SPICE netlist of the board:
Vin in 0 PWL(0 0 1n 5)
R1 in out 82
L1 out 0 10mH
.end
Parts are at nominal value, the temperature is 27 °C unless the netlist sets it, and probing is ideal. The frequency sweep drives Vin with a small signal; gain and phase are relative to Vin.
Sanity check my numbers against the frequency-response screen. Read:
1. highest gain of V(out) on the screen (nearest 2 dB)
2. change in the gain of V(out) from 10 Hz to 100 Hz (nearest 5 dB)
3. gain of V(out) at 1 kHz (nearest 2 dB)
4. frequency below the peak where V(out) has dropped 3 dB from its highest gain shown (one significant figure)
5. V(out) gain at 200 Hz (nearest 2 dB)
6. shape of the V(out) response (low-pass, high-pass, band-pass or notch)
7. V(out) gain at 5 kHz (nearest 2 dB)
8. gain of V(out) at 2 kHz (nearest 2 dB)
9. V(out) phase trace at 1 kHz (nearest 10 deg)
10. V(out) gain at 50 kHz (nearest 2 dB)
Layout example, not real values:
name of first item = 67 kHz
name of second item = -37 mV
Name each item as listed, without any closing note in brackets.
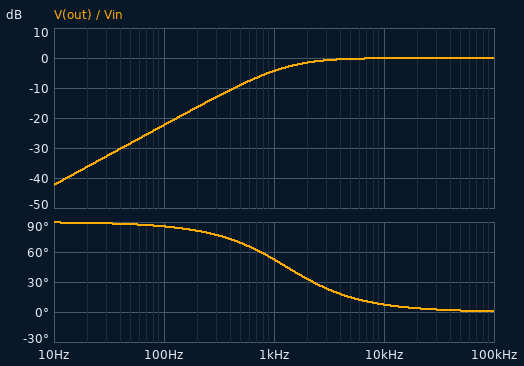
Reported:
highest gain of V(out) on the screen = 0 dB
change in the gain of V(out) from 10 Hz to 100 Hz = 20 dB
gain of V(out) at 1 kHz = -4 dB
frequency below the peak where V(out) has dropped 3 dB from its highest gain shown = 1 kHz
V(out) gain at 200 Hz = -16 dB
shape of the V(out) response = high-pass
V(out) gain at 5 kHz = 0 dB
gain of V(out) at 2 kHz = -2 dB
V(out) phase trace at 1 kHz = 50 deg
V(out) gain at 50 kHz = 0 dB
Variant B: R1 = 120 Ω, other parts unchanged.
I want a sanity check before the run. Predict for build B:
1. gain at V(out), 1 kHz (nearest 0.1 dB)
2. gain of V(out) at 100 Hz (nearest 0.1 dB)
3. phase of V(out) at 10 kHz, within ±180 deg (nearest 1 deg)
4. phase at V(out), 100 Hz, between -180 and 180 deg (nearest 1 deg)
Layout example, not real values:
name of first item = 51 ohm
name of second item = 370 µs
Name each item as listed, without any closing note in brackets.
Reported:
gain at V(out), 1 kHz = -6.7 dB
gain of V(out) at 100 Hz = -25.6 dB
phase of V(out) at 10 kHz, within ±180 deg = 11 deg
phase at V(out), 100 Hz, between -180 and 180 deg = 87 deg
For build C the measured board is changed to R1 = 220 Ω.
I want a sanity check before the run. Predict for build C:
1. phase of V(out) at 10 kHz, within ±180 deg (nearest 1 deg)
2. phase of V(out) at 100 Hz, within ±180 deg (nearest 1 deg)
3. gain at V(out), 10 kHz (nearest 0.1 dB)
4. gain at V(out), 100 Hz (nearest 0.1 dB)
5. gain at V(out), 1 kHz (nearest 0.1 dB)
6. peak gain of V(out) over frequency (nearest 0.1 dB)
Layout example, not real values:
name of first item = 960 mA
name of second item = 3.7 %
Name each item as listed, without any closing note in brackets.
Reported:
phase of V(out) at 10 kHz, within ±180 deg = 19 deg
phase of V(out) at 100 Hz, within ±180 deg = 88 deg
gain at V(out), 10 kHz = -0.5 dB
gain at V(out), 100 Hz = -30.9 dB
gain at V(out), 1 kHz = -11.2 dB
peak gain of V(out) over frequency = 0 dB
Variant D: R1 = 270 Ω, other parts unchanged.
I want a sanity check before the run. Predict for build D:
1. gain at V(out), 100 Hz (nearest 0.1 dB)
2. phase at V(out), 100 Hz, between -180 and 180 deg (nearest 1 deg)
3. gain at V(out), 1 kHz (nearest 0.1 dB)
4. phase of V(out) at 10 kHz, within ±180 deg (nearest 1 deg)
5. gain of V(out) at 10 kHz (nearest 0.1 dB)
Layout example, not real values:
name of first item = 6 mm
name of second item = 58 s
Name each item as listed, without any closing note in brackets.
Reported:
gain at V(out), 100 Hz = -32.7 dB
phase at V(out), 100 Hz, between -180 and 180 deg = 89 deg
gain at V(out), 1 kHz = -12.9 dB
phase of V(out) at 10 kHz, within ±180 deg = 23 deg
gain of V(out) at 10 kHz = -0.7 dB
